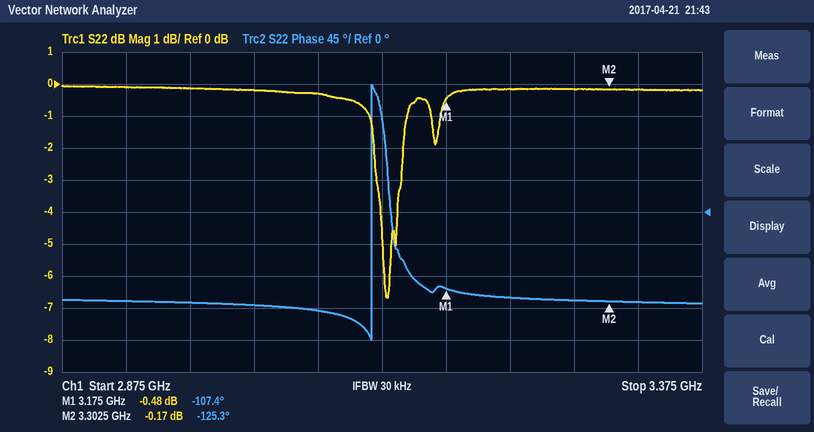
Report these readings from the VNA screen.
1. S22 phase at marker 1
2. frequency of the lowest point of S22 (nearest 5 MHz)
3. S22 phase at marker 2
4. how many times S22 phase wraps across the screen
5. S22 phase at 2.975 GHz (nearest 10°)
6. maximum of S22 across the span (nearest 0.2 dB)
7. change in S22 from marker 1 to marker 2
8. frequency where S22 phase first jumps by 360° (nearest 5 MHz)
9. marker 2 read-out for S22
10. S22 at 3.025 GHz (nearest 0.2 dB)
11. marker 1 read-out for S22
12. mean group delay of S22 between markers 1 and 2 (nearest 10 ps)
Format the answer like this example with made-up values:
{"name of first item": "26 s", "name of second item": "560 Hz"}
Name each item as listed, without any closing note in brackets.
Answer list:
{"S22 phase at marker 1": "-107.4°", "frequency of the lowest point of S22": "3.130 GHz", "S22 phase at marker 2": "-125.3°", "how many times S22 phase wraps across the screen": "1", "S22 phase at 2.975 GHz": "-130°", "maximum of S22 across the span": "0.0 dB", "change in S22 from marker 1 to marker 2": "0.31 dB", "frequency where S22 phase first jumps by 360°": "3.115 GHz", "marker 2 read-out for S22": "-0.17 dB", "S22 at 3.025 GHz": "-0.2 dB", "marker 1 read-out for S22": "-0.48 dB", "mean group delay of S22 between markers 1 and 2": "390 ps"}
